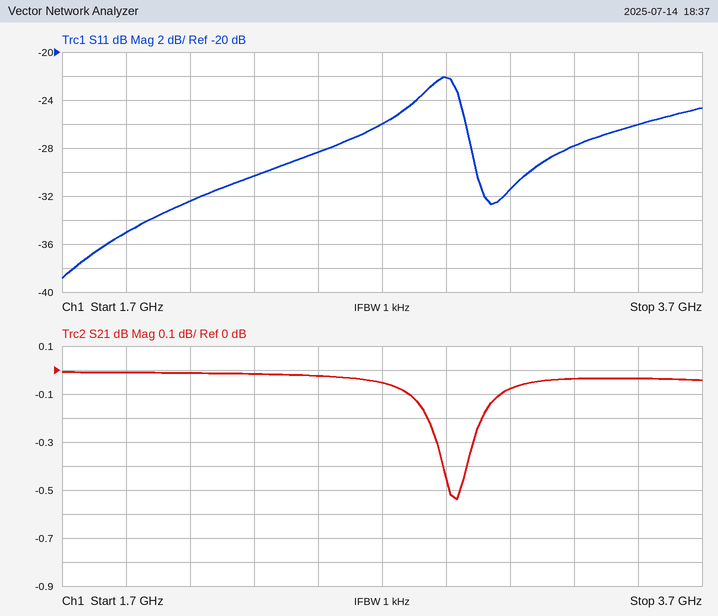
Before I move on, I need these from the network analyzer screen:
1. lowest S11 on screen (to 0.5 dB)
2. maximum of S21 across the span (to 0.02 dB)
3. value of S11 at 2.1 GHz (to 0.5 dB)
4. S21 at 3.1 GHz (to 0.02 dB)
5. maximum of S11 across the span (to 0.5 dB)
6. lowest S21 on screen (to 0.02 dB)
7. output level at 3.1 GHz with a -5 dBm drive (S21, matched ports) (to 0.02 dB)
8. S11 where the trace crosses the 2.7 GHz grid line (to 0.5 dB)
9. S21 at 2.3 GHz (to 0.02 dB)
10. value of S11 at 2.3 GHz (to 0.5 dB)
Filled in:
-39.0 dB
0.00 dB
-32.5 dB
-0.08 dB
-22.0 dB
-0.54 dB
-5.08 dBm
-26.0 dB
-0.02 dB
-30.5 dB
